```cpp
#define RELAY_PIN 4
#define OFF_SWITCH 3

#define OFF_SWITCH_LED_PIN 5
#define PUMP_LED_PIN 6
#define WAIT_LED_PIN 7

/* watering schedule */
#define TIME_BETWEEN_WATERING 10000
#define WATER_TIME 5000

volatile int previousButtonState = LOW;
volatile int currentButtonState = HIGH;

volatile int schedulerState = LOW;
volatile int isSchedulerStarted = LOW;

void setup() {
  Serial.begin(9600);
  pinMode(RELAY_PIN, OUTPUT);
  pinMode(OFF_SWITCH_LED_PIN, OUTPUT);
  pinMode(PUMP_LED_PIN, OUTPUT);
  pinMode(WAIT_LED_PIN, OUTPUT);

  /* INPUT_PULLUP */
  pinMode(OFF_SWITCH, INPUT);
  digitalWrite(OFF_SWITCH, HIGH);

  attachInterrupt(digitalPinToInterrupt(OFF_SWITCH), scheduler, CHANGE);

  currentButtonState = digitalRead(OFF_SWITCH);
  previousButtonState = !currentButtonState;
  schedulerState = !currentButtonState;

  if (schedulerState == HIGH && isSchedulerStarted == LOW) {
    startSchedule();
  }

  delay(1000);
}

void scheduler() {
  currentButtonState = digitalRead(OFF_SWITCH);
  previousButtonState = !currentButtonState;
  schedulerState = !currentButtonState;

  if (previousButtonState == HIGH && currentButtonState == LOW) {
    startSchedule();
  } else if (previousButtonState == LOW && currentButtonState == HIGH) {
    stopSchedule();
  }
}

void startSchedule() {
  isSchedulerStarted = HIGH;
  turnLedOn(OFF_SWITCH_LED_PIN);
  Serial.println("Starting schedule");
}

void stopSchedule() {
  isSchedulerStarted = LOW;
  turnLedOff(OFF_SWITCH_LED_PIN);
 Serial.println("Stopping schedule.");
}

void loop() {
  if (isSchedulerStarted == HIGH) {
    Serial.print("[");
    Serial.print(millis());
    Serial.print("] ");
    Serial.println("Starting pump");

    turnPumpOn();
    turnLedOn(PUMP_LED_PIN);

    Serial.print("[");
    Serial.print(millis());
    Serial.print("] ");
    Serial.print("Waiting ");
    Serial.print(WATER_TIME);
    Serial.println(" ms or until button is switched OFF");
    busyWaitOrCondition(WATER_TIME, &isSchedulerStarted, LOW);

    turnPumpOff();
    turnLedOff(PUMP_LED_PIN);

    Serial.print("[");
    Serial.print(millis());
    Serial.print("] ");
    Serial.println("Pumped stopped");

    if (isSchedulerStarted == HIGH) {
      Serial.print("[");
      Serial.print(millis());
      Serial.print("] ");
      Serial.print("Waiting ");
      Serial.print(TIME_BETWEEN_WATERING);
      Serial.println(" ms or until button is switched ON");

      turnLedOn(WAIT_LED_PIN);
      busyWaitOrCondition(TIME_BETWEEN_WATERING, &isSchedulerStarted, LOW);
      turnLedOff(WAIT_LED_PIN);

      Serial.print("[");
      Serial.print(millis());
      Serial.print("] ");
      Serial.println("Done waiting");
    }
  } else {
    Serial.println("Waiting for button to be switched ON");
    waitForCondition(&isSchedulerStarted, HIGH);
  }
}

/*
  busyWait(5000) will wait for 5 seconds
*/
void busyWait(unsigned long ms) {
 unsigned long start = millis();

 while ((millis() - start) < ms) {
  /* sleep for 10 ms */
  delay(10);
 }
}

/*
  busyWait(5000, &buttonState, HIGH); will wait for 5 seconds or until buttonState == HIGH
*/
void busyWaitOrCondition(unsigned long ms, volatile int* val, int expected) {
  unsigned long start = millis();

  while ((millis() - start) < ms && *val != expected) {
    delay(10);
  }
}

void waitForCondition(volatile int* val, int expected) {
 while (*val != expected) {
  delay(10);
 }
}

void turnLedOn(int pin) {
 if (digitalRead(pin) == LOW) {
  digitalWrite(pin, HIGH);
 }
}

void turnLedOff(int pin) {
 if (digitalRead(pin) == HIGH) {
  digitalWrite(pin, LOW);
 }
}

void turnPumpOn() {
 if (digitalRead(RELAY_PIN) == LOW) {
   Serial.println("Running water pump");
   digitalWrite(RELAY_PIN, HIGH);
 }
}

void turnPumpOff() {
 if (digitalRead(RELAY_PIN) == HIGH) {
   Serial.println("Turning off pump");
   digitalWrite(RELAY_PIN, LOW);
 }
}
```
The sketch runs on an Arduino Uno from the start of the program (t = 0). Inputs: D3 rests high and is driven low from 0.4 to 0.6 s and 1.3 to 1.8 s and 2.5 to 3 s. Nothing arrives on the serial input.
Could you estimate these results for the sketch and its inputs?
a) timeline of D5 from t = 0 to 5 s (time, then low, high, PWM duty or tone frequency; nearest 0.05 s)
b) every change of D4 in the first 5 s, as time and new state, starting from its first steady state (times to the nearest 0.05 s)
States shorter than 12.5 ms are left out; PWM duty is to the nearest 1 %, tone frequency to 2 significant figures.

0 s low; 0.4 s high; 0.6 s low; 1.3 s high; 1.8 s low; 2.5 s high; 3 s low
0 s low; 1.3 s high; 1.8 s low; 2.5 s high; 3 s low
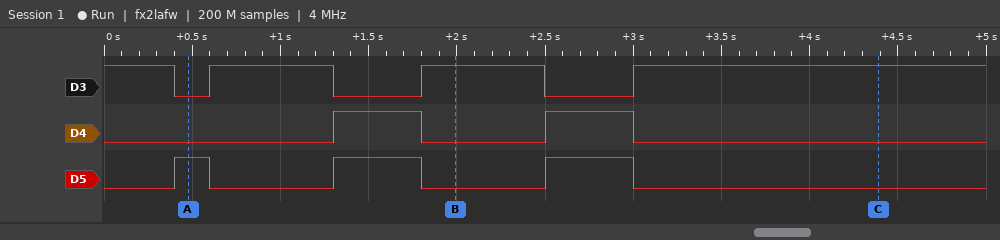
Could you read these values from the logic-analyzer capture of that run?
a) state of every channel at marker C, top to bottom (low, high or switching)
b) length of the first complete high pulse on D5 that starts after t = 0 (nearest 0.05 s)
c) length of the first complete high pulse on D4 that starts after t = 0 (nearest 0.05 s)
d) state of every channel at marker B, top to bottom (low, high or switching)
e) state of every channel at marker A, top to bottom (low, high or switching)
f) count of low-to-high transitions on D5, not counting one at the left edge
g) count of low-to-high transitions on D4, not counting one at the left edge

D3 high, D4 low, D5 low
0.20 s
0.50 s
D3 high, D4 low, D5 low
D3 low, D4 low, D5 high
3
2
